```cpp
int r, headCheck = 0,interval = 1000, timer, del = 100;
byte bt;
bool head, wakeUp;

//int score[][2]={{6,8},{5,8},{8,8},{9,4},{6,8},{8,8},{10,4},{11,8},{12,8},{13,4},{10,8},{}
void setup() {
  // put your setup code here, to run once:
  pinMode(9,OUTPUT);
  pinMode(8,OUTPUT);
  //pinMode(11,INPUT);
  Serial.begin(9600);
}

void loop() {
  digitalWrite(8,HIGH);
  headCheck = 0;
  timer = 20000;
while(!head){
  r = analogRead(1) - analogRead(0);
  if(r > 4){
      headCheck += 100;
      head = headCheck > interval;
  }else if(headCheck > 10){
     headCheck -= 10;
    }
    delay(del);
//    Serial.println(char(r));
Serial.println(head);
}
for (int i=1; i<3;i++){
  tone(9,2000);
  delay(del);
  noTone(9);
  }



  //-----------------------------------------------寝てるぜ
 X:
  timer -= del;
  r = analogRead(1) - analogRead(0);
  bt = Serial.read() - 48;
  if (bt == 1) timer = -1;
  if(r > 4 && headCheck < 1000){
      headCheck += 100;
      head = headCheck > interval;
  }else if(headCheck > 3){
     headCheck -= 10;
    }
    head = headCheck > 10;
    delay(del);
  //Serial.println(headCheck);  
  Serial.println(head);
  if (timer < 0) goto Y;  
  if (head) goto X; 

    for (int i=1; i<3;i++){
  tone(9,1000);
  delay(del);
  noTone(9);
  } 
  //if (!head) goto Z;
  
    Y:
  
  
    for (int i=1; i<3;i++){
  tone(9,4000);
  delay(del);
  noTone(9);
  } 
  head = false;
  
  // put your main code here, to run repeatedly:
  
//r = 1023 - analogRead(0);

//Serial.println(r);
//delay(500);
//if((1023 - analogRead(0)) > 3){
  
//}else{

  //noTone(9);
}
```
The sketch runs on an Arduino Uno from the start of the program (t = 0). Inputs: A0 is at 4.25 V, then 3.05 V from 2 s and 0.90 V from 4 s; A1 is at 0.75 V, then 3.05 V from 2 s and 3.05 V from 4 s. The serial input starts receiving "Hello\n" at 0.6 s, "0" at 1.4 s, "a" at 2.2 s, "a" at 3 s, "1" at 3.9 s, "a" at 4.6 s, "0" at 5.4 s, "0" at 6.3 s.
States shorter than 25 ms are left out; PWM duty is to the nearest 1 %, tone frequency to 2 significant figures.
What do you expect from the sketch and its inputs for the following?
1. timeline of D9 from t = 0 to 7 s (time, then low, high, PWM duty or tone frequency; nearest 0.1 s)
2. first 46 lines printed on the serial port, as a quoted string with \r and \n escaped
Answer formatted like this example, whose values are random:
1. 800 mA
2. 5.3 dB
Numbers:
1. 0 s low; 5.1 s tone 2000 Hz; 5.3 s low; 6.3 s tone 4000 Hz; 6.5 s low
2. "0\r\n0\r\n0\r\n0\r\n0\r\n0\r\n0\r\n0\r\n0\r\n0\r\n0\r\n0\r\n0\r\n0\r\n0\r\n0\r\n0\r\n0\r\n0\r\n0\r\n0\r\n0\r\n0\r\n0\r\n0\r\n0\r\n0\r\n0\r\n0\r\n0\r\n0\r\n0\r\n0\r\n0\r\n0\r\n0\r\n0\r\n0\r\n0\r\n0\r\n0\r\n0\r\n0\r\n0\r\n0\r\n0\r\n"
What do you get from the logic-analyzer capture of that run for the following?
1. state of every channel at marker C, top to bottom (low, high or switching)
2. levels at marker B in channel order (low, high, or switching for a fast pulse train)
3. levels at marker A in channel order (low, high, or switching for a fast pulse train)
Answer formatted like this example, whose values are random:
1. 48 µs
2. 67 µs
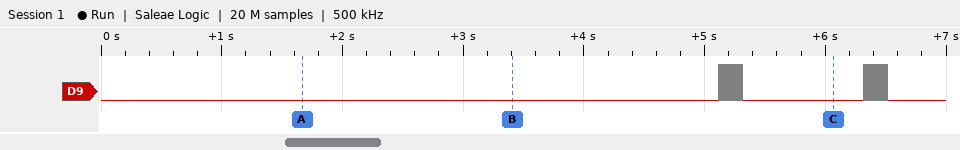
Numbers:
1. D9 low
2. D9 low
3. D9 low
